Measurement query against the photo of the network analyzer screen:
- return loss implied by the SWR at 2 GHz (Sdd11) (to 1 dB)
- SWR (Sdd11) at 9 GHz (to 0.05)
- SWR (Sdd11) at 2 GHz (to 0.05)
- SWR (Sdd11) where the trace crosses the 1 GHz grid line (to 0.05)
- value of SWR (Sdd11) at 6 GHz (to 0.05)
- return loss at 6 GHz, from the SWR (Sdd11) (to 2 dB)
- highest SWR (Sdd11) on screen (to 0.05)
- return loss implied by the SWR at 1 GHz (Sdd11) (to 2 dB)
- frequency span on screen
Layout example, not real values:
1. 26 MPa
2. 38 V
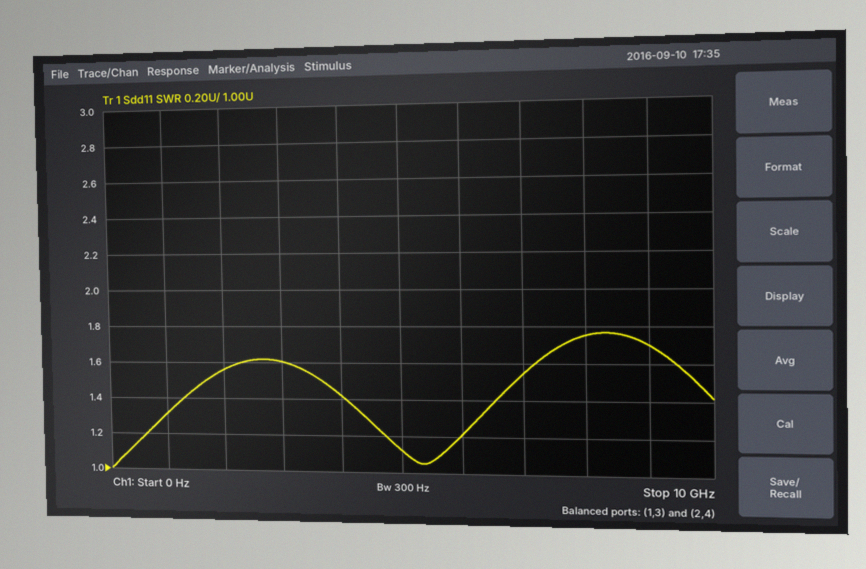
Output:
1. 13 dB
2. 1.70
3. 1.55
4. 1.30
5. 1.20
6. 20 dB
7. 1.75
8. 18 dB
9. 10 GHz
